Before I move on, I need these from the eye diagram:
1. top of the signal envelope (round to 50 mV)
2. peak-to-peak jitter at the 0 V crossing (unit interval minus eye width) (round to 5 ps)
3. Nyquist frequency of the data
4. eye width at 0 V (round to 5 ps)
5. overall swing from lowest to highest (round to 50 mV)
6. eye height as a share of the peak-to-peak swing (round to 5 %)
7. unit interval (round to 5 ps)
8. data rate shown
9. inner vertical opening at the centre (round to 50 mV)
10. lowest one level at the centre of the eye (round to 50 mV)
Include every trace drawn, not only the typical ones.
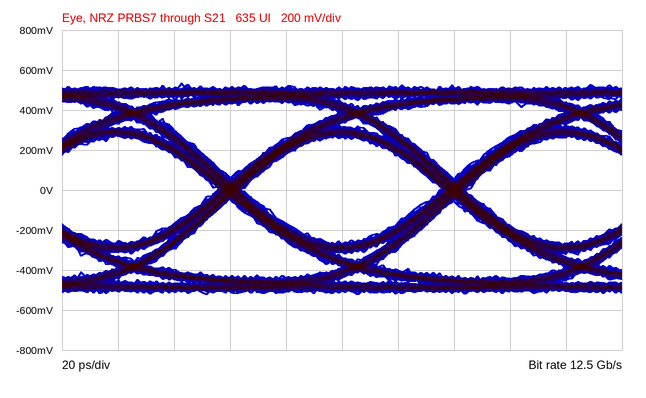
550 mV
10 ps
6.25 GHz
70 ps
1.05 V
50 %
80 ps
12.5 Gb/s
550 mV
250 mV
